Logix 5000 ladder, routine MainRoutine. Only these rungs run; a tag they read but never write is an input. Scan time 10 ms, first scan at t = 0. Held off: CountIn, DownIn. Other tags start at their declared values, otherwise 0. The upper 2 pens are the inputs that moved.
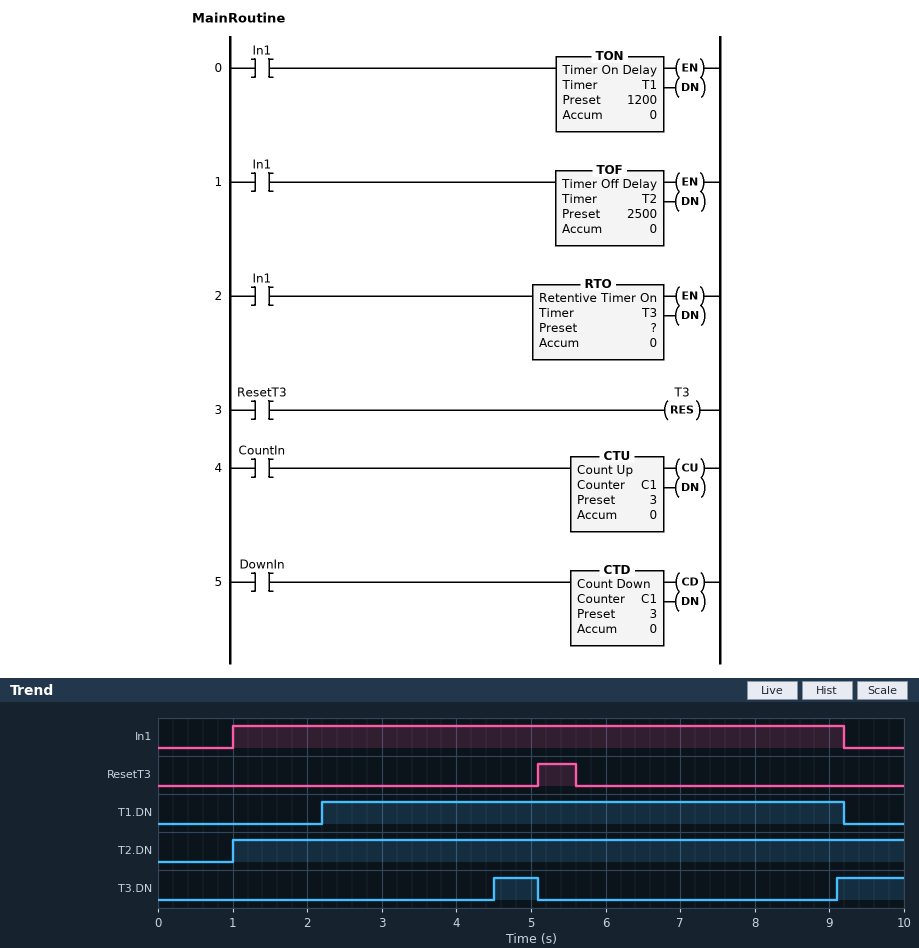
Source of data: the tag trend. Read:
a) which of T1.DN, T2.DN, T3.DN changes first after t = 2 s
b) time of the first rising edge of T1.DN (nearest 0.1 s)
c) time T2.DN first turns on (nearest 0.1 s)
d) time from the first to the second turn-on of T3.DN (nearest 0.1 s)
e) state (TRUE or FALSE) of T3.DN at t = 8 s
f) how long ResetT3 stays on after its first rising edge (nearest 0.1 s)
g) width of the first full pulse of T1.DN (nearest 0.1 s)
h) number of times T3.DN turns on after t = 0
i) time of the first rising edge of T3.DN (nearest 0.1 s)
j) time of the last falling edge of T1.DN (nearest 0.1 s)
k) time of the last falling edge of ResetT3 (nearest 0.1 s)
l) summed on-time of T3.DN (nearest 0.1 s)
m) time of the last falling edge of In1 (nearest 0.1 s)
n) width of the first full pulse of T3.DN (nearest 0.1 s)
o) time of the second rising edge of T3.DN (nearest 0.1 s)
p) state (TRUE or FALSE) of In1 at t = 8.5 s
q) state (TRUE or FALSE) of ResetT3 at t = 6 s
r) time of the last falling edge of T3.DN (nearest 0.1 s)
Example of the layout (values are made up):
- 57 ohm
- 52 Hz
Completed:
- T1.DN
- 2.2 s
- 1.0 s
- 4.6 s
- FALSE
- 0.5 s
- 7.0 s
- 2
- 4.5 s
- 9.2 s
- 5.6 s
- 1.5 s
- 9.2 s
- 0.6 s
- 9.1 s
- TRUE
- FALSE
- 5.1 s
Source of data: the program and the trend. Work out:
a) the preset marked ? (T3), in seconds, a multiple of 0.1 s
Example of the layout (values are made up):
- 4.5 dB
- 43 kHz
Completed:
- 3.5 s
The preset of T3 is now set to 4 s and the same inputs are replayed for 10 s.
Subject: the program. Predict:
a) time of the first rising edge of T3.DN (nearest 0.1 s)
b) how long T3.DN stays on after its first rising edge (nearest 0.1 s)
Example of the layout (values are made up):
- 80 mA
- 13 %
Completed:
- 5.0 s
- 0.1 s
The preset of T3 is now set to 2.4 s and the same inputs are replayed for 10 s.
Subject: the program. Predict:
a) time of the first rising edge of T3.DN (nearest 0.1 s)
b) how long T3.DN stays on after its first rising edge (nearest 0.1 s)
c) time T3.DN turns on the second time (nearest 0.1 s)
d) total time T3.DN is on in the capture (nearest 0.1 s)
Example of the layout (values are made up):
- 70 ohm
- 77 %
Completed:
- 3.4 s
- 1.7 s
- 8.0 s
- 3.7 s
